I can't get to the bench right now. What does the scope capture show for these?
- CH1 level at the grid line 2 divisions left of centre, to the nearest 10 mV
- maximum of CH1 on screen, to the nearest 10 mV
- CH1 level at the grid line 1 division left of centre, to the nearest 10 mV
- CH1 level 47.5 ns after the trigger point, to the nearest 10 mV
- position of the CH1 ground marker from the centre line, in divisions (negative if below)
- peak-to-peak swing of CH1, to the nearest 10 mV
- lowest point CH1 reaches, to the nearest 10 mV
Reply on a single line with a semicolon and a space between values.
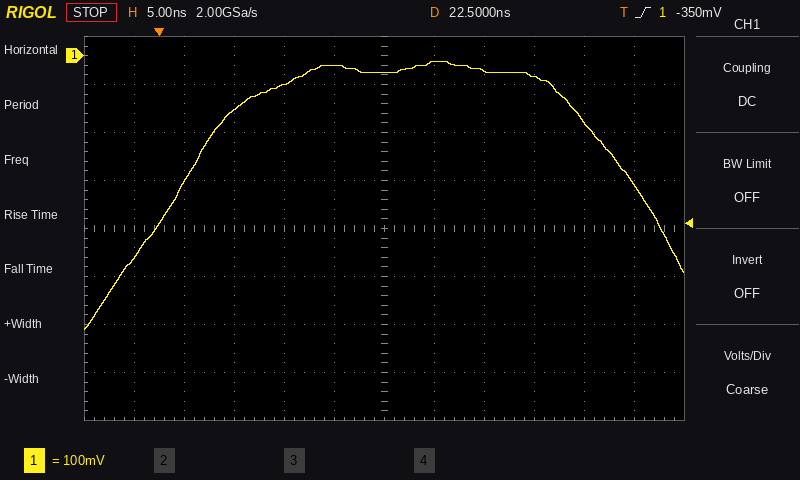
-60 mV; -10 mV; -20 mV; -270 mV; +3.6 div; 560 mV; -570 mV
